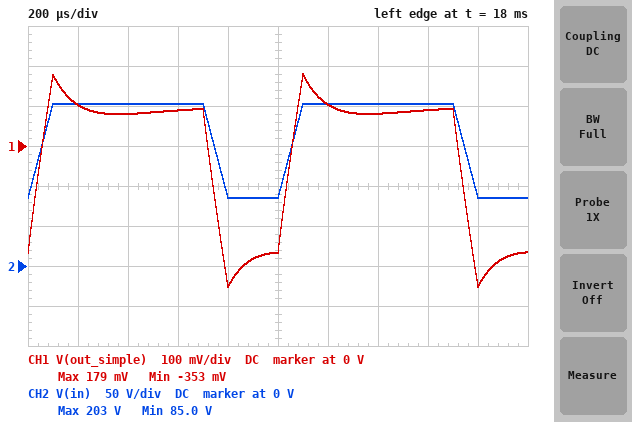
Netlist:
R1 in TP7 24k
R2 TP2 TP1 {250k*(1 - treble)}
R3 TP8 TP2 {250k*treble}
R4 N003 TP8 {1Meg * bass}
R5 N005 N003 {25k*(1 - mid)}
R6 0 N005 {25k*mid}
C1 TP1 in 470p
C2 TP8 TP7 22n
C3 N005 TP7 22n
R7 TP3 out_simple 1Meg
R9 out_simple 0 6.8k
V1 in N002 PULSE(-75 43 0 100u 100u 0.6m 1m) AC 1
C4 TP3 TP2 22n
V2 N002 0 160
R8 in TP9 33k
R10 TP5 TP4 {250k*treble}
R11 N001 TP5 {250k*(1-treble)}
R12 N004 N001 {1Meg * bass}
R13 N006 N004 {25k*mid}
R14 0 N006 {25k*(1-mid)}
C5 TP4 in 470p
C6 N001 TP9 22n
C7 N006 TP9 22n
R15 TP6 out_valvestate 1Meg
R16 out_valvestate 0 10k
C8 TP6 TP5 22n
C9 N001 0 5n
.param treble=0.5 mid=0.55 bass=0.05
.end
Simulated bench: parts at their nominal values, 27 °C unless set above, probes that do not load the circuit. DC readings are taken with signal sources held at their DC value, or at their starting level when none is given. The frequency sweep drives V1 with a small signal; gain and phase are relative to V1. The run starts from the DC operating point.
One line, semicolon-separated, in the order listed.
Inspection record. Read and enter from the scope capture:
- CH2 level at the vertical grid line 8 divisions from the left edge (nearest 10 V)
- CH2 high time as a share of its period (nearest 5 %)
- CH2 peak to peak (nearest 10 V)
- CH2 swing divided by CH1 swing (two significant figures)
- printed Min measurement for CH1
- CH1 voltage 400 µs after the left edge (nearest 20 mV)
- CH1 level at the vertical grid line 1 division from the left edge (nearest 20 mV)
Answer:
200 V; 70 %; 120 V; 220; -353 mV; 80 mV; 100 mV
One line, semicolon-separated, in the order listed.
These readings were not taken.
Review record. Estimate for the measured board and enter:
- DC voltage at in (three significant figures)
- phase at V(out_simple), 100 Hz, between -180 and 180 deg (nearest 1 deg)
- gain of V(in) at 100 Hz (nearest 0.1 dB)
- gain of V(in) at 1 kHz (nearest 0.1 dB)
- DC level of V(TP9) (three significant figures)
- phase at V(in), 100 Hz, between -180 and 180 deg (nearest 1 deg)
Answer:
85.0 V; 30 deg; 0 dB; 0 dB; 85.0 V; 0 deg
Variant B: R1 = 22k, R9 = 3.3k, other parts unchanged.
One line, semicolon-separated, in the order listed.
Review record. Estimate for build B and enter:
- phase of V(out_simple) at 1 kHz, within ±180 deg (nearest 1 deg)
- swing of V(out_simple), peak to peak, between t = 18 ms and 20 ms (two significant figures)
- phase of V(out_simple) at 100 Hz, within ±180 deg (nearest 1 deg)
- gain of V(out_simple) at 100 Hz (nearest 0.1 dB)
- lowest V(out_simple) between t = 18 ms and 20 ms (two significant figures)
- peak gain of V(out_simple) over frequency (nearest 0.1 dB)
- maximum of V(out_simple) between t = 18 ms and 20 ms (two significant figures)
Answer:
8 deg; 260 mV; 31 deg; -54.5 dB; -170 mV; -53.3 dB; 87 mV
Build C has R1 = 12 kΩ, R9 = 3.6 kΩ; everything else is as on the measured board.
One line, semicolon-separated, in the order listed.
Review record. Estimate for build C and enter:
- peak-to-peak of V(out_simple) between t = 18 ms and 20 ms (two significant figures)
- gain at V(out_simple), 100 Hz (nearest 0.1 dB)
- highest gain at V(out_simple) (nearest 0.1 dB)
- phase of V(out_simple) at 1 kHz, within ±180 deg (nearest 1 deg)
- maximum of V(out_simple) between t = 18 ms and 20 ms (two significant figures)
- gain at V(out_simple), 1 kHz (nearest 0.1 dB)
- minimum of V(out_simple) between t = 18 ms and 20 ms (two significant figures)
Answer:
310 mV; -52.7 dB; -51.7 dB; 4 deg; 94 mV; -53.4 dB; -210 mV
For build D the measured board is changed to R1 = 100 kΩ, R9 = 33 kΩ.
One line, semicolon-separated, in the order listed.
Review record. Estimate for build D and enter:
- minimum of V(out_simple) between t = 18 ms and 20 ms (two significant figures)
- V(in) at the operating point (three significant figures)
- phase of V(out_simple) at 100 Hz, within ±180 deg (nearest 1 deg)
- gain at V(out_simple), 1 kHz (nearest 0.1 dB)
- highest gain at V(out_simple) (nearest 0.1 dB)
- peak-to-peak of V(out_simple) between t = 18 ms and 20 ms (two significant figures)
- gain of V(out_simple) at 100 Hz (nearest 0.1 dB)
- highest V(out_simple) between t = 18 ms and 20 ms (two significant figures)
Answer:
-1.4 V; 85.0 V; 14 deg; -39.9 dB; -35.2 dB; 2.4 V; -41.2 dB; 970 mV
